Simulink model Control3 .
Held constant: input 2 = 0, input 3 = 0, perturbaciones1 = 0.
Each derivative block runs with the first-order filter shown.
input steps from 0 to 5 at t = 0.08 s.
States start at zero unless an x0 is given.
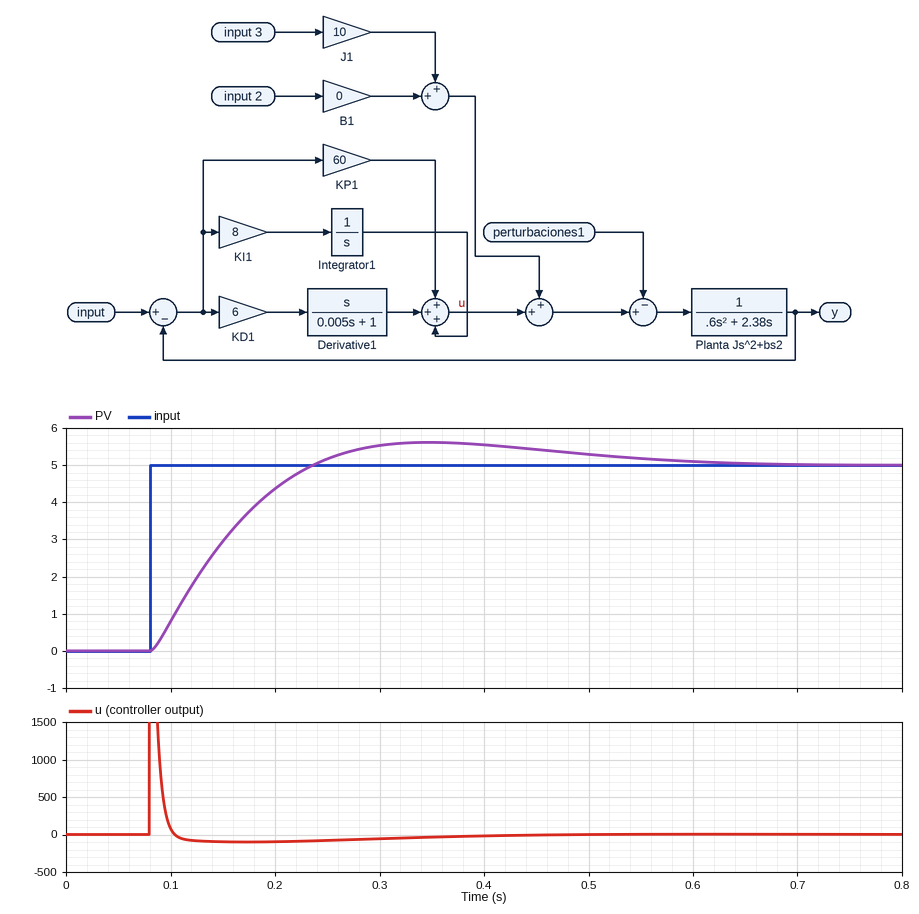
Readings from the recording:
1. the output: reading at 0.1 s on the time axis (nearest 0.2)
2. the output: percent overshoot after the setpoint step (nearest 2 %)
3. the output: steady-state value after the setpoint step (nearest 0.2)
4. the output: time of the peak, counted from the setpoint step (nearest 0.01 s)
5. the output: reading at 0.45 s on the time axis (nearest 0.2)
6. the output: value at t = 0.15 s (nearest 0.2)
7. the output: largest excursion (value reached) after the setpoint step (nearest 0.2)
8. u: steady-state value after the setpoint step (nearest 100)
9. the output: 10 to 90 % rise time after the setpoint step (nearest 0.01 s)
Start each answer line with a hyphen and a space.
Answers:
- 0.8
- 12 %
- 5.0
- 0.27 s
- 5.4
- 3.0
- 5.6
- 0
- 0.11 s
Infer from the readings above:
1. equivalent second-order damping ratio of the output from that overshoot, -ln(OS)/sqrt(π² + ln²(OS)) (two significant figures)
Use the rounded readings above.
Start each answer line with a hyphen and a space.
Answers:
- 0.56
